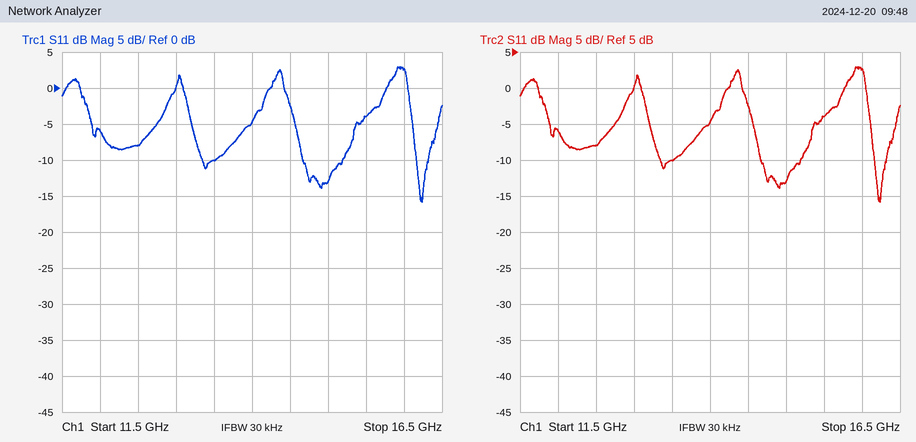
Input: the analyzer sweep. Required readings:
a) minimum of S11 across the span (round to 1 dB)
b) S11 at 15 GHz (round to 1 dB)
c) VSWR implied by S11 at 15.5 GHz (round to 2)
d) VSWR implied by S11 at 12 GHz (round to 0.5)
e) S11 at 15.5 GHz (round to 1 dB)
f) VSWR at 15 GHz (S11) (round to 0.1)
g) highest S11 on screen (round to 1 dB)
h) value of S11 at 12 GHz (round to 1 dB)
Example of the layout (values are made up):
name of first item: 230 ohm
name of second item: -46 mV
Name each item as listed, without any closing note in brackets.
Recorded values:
minimum of S11 across the span: -16 dB
S11 at 15 GHz: -13 dB
VSWR implied by S11 at 15.5 GHz: 4
VSWR implied by S11 at 12 GHz: 3.0
S11 at 15.5 GHz: -4 dB
VSWR at 15 GHz (S11): 1.6
highest S11 on screen: 3 dB
value of S11 at 12 GHz: -6 dB
